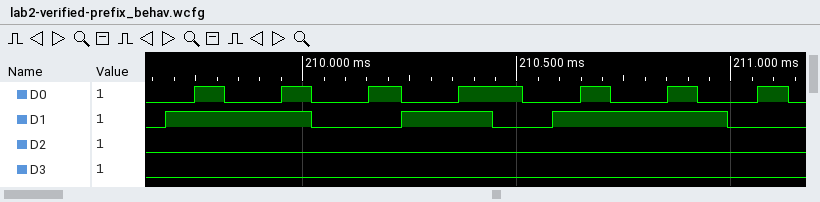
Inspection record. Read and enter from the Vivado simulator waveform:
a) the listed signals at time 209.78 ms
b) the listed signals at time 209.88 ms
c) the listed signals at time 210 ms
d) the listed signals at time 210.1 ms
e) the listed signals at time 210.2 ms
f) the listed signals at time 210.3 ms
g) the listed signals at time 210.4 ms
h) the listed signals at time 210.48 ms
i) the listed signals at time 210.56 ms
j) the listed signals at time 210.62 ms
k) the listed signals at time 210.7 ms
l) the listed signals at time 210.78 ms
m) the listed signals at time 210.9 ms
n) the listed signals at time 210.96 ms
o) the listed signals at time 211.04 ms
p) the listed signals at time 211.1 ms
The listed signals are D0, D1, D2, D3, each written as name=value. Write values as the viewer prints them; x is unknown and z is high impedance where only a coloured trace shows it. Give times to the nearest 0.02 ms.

D0=1, D1=1, D2=0, D3=0
D0=0, D1=1, D2=0, D3=0
D0=1, D1=1, D2=0, D3=0
D0=0, D1=0, D2=0, D3=0
D0=1, D1=0, D2=0, D3=0
D0=0, D1=1, D2=0, D3=0
D0=1, D1=1, D2=0, D3=0
D0=1, D1=0, D2=0, D3=0
D0=0, D1=0, D2=0, D3=0
D0=0, D1=1, D2=0, D3=0
D0=1, D1=1, D2=0, D3=0
D0=0, D1=1, D2=0, D3=0
D0=1, D1=1, D2=0, D3=0
D0=0, D1=1, D2=0, D3=0
D0=0, D1=0, D2=0, D3=0
D0=1, D1=0, D2=0, D3=0
